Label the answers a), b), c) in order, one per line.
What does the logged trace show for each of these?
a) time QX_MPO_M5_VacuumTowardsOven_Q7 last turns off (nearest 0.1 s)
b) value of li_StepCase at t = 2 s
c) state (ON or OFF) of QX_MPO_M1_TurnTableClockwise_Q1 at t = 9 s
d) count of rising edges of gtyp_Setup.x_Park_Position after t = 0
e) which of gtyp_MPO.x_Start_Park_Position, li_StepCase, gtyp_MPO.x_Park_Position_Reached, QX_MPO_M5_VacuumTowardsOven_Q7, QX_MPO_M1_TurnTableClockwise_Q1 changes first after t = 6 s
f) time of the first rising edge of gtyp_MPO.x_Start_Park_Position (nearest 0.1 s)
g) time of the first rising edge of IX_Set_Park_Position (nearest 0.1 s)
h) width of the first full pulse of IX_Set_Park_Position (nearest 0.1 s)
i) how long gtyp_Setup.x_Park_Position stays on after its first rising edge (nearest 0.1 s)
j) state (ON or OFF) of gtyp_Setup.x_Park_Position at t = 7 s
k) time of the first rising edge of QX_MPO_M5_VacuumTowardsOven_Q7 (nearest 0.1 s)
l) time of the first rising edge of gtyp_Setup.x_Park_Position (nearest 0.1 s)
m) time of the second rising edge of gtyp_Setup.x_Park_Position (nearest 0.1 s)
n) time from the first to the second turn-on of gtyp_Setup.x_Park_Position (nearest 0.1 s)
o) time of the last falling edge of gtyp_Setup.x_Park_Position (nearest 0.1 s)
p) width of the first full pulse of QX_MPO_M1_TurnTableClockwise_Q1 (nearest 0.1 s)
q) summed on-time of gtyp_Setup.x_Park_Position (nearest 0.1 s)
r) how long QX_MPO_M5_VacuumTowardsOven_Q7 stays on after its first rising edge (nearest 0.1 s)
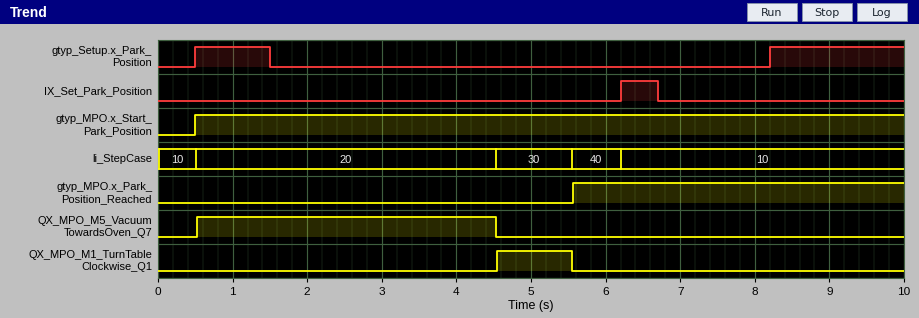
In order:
a) 4.5 s
b) 20
c) OFF
d) 2
e) li_StepCase
f) 0.5 s
g) 6.2 s
h) 0.5 s
i) 1.0 s
j) OFF
k) 0.5 s
l) 0.5 s
m) 8.2 s
n) 7.7 s
o) 1.5 s
p) 1.0 s
q) 2.8 s
r) 4.0 s
